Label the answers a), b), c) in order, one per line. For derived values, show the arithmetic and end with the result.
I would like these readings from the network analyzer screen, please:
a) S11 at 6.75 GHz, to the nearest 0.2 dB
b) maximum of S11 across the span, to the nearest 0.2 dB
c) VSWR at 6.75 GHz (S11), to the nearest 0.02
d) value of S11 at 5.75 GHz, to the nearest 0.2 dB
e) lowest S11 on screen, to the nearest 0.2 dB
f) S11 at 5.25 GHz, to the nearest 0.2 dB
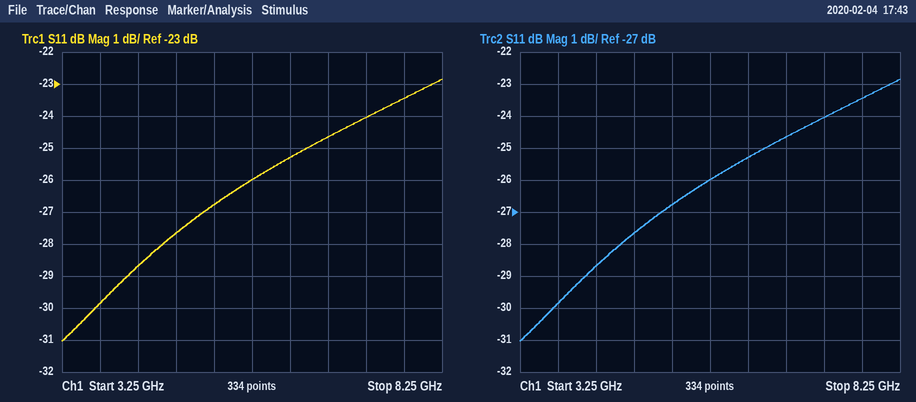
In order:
a) -24.6 dB
b) -22.8 dB
c) |Γ| = 10^(-24.6/20) = 0.0589; VSWR = (1 + 0.0589)/(1 − 0.0589) ≈ 1.13, so 1.12 to the nearest 0.02
d) -26.0 dB
e) -31.0 dB
f) -26.8 dB
